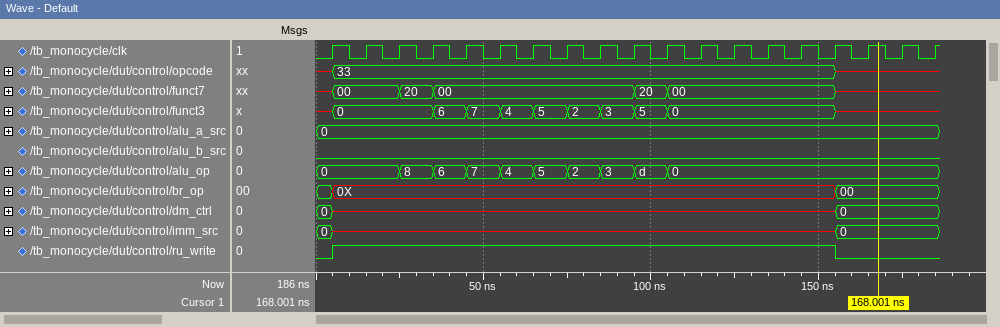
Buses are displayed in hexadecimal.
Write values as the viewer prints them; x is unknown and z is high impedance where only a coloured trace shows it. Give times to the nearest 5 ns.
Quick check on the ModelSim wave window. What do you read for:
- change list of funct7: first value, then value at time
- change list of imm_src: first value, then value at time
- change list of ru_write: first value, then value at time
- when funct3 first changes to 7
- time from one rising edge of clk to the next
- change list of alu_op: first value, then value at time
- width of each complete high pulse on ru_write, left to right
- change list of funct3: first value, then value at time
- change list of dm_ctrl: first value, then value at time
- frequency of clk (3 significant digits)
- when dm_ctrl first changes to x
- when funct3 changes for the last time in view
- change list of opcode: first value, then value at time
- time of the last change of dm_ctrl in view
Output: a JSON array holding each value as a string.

["x, 00 at 5 ns, 20 at 25 ns, 00 at 35 ns, 20 at 95 ns, 00 at 105 ns, x at 155 ns", "0, x at 5 ns, 0 at 155 ns", "0, 1 at 5 ns, 0 at 155 ns", "45 ns", "10 ns", "0, 8 at 25 ns, 6 at 35 ns, 7 at 45 ns, 4 at 55 ns, 5 at 65 ns, 2 at 75 ns, 3 at 85 ns, d at 95 ns, 0 at 105 ns", "150 ns", "x, 0 at 5 ns, 6 at 35 ns, 7 at 45 ns, 4 at 55 ns, 5 at 65 ns, 2 at 75 ns, 3 at 85 ns, 5 at 95 ns, 0 at 105 ns, x at 155 ns", "0, x at 5 ns, 0 at 155 ns", "100 MHz", "5 ns", "155 ns", "x, 33 at 5 ns, x at 155 ns", "155 ns"]
